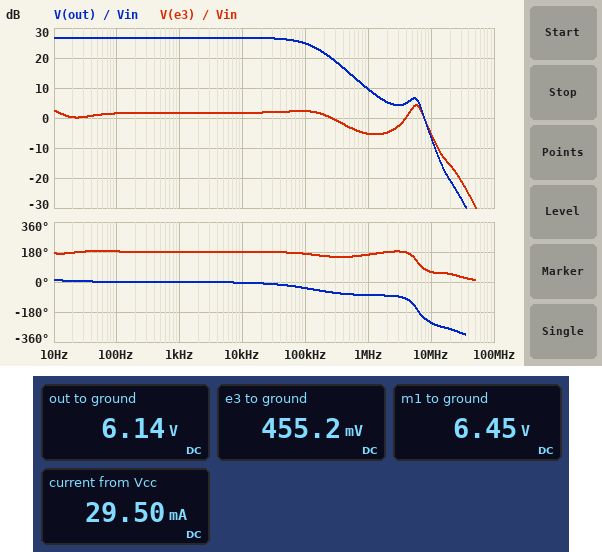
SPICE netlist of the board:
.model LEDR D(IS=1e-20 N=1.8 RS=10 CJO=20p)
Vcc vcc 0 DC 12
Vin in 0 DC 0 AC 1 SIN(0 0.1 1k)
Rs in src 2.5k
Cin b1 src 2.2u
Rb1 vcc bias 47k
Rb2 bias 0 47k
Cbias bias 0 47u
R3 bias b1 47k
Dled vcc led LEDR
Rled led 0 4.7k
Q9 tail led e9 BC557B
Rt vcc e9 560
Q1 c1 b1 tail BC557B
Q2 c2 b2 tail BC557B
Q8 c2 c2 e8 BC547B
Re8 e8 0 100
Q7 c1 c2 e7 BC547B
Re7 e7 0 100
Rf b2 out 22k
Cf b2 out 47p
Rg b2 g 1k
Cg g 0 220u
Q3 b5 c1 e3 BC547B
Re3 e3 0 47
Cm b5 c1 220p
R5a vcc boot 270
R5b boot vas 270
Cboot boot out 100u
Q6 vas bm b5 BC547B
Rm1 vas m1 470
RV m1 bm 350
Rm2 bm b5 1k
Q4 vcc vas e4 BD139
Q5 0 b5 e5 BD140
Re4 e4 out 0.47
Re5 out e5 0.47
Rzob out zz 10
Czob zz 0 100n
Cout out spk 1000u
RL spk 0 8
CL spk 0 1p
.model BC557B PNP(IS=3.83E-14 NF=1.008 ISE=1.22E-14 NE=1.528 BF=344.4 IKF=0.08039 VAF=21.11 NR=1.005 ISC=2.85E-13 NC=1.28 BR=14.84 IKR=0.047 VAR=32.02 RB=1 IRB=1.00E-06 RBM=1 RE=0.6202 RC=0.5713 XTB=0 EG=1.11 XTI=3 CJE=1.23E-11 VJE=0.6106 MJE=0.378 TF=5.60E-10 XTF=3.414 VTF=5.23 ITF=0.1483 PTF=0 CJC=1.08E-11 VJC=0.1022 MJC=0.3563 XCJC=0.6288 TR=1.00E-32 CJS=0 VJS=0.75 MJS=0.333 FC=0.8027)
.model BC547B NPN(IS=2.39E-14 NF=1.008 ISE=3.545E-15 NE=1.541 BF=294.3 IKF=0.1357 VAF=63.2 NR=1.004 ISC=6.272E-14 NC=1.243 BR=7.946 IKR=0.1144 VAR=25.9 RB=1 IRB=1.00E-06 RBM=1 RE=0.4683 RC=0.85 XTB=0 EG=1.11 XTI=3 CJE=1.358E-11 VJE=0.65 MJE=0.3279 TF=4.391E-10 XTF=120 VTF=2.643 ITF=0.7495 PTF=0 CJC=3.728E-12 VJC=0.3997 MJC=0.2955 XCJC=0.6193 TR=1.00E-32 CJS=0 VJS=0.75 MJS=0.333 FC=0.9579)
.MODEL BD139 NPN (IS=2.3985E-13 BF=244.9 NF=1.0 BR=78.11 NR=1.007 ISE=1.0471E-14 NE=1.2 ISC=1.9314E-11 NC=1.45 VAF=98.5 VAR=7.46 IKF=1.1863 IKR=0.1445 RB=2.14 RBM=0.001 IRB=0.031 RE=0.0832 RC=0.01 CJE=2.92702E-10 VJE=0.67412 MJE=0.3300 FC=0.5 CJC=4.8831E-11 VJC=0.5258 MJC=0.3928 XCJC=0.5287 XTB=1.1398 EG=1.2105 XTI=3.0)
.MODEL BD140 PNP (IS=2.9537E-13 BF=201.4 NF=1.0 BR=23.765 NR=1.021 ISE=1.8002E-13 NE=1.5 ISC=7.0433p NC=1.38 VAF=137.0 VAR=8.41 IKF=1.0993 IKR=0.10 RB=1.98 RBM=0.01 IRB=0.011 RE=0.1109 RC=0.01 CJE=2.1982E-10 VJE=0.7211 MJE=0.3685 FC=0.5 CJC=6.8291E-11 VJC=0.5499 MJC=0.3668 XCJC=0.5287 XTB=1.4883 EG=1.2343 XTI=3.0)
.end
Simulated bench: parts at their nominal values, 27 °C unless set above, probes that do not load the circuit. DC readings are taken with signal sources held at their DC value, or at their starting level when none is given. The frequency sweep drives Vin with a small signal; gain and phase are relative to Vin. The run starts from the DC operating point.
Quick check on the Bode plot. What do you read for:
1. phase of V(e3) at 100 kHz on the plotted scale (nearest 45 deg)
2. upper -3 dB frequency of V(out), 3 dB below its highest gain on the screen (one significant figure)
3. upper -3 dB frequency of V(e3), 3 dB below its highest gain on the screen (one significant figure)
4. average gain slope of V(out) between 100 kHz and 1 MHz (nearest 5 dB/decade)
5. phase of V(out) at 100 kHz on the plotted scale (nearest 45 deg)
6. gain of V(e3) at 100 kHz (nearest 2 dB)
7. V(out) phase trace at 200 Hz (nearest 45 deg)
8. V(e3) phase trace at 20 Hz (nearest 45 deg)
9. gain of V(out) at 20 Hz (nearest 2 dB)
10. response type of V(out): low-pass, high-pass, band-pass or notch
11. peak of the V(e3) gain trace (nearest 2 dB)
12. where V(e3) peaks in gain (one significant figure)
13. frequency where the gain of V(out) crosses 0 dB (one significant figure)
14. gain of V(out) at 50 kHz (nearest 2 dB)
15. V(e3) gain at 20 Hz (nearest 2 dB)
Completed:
180 deg
100 kHz
7 MHz
-15 dB/decade
-45 deg
2 dB
0 deg
180 deg
26 dB
low-pass
4 dB
6 MHz
8 MHz
26 dB
0 dB
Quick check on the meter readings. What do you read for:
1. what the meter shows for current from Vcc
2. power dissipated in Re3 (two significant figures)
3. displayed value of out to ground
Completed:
29.50 mA
4.4 mW
6.14 V
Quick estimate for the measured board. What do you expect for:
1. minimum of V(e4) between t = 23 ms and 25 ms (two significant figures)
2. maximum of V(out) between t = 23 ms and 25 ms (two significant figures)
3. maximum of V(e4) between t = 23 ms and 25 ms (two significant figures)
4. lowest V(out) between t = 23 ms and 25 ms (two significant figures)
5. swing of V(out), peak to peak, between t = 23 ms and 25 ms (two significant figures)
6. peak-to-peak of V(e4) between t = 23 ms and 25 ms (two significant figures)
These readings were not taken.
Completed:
4.0 V
8.3 V
8.4 V
4.0 V
4.3 V
4.5 V
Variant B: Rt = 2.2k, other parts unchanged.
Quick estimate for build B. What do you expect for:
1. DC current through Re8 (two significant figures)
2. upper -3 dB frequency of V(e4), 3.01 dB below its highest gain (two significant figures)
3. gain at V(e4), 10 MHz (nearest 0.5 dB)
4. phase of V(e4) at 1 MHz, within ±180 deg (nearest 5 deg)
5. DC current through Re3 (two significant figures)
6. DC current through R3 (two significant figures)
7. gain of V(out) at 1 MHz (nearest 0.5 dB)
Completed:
270 µA
100 kHz
-15.5 dB
-90 deg
9.9 mA
770 nA
7.0 dB
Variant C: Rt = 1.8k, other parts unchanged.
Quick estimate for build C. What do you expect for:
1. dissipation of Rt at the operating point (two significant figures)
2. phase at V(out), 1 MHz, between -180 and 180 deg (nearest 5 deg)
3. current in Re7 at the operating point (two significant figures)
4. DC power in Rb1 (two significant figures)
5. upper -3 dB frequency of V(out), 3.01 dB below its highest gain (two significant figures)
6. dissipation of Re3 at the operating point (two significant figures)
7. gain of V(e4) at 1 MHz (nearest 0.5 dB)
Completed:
890 µW
-90 deg
330 µA
760 µW
110 kHz
4.6 mW
8.0 dB
